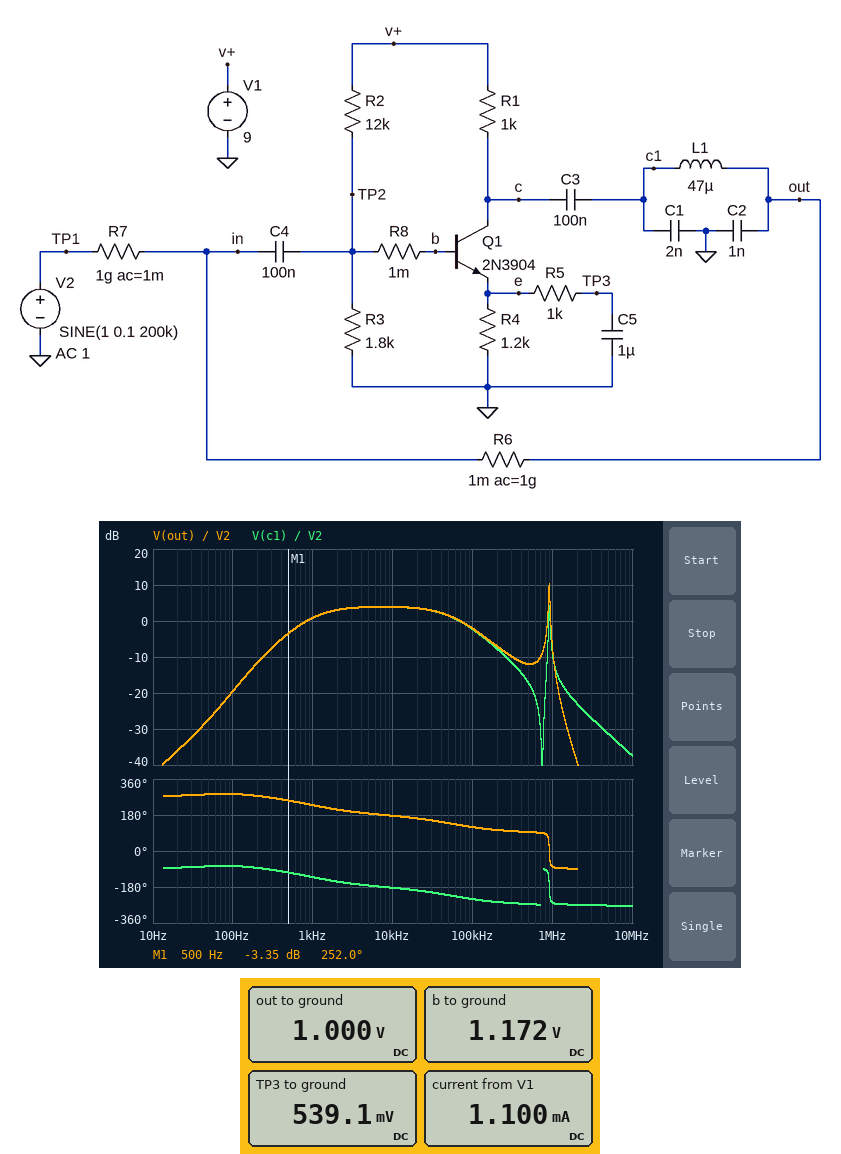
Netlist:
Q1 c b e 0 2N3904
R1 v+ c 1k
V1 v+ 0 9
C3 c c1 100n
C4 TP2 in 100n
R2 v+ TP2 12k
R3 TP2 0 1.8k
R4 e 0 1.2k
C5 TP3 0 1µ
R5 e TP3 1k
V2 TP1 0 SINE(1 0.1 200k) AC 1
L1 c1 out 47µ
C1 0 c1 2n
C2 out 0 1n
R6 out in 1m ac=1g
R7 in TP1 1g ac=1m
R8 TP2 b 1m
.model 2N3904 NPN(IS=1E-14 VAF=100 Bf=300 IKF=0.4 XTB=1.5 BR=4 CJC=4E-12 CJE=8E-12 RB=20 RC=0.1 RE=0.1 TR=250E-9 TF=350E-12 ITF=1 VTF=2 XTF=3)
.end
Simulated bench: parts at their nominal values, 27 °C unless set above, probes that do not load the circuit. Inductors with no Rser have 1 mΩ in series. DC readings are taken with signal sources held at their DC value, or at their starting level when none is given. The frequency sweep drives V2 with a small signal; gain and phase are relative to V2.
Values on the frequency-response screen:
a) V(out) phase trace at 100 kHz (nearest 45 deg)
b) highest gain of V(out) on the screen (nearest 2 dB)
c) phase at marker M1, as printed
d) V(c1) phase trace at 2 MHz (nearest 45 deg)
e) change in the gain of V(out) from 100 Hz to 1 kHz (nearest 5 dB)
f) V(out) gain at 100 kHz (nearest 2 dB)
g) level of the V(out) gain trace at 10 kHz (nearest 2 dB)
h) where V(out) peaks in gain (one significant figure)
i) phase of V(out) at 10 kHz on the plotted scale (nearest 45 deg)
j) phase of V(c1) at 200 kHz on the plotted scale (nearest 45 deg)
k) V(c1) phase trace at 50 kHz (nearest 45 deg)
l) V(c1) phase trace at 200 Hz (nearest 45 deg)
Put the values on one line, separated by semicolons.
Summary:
135 deg; 10 dB; 252.0 deg; -270 deg; 20 dB; -2 dB; 4 dB; 900 kHz; 180 deg; -270 deg; -225 deg; -90 deg
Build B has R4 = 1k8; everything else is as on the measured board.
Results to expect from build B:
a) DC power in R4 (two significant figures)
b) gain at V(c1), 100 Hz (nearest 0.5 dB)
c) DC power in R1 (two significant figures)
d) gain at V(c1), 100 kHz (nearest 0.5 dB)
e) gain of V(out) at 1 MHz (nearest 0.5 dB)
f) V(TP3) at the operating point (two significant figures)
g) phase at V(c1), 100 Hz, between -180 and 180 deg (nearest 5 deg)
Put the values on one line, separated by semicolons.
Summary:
170 µW; -21.5 dB; 93 µW; -4.0 dB; -10.5 dB; 550 mV; -70 deg
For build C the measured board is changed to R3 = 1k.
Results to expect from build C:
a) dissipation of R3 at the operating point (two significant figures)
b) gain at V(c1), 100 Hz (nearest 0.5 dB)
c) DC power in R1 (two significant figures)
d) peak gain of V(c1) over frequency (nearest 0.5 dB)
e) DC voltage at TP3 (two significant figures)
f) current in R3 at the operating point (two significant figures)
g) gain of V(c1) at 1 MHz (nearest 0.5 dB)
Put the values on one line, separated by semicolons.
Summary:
480 µW; -26.0 dB; 7.3 µW; 1.5 dB; 100 mV; 690 µA; -13.0 dB
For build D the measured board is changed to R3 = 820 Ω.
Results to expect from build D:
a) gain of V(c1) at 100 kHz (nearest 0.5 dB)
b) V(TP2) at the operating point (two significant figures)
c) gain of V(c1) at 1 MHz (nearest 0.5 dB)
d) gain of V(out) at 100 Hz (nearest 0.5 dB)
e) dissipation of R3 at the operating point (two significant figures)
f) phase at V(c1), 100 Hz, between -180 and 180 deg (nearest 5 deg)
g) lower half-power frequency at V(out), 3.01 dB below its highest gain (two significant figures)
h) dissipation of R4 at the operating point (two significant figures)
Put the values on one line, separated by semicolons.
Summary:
-12.0 dB; 580 mV; -20.0 dB; -33.0 dB; 400 µW; -85 deg; 880 kHz; 480 nW
